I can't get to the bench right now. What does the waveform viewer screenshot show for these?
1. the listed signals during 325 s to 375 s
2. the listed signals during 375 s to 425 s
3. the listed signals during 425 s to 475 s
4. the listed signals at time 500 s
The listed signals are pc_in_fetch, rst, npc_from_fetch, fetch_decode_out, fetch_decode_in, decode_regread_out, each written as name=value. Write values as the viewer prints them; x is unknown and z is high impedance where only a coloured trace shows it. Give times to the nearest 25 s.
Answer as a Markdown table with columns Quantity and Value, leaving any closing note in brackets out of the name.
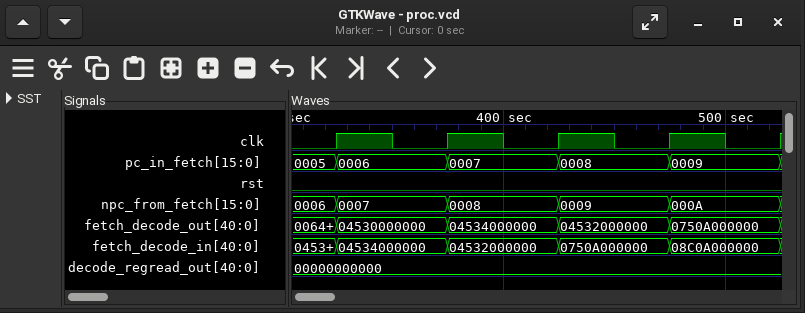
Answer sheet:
| Quantity | Value |
|---|---|
| the listed signals during 325 s to 375 s | pc_in_fetch=0006, rst=0, npc_from_fetch=0007, fetch_decode_out=04530000000, fetch_decode_in=04534000000, decode_regread_out=00000000000 |
| the listed signals during 375 s to 425 s | pc_in_fetch=0007, rst=0, npc_from_fetch=0008, fetch_decode_out=04534000000, fetch_decode_in=04532000000, decode_regread_out=00000000000 |
| the listed signals during 425 s to 475 s | pc_in_fetch=0008, rst=0, npc_from_fetch=0009, fetch_decode_out=04532000000, fetch_decode_in=0750A000000, decode_regread_out=00000000000 |
| the listed signals at time 500 s | pc_in_fetch=0009, rst=0, npc_from_fetch=000A, fetch_decode_out=0750A000000, fetch_decode_in=08C0A000000, decode_regread_out=00000000000 |
